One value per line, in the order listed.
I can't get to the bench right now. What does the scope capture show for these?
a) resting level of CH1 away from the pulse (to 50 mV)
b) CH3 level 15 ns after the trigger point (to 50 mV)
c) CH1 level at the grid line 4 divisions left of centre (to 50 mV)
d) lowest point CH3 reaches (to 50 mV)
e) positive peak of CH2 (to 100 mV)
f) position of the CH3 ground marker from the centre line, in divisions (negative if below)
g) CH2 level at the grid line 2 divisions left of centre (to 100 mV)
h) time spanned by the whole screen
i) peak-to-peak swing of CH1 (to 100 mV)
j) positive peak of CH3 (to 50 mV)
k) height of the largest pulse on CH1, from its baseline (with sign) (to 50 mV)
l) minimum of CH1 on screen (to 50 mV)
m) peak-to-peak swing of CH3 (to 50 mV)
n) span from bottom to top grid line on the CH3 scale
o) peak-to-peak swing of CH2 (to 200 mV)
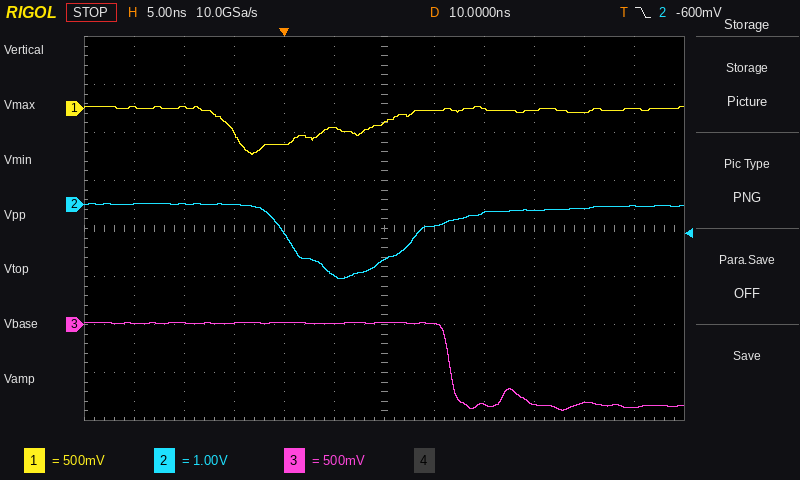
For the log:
0 mV
0 mV
0 mV
-900 mV
0.0 V
-2.0 div
-600 mV
60 ns
500 mV
0 mV
-500 mV
-500 mV
900 mV
4 V
1.6 V
